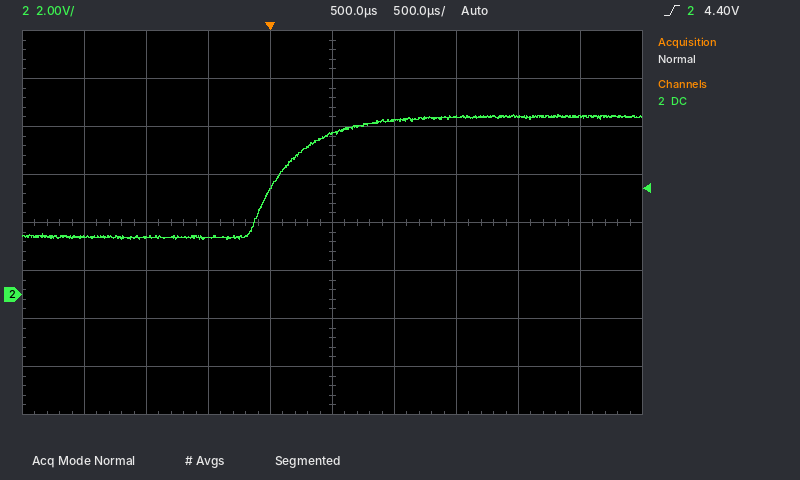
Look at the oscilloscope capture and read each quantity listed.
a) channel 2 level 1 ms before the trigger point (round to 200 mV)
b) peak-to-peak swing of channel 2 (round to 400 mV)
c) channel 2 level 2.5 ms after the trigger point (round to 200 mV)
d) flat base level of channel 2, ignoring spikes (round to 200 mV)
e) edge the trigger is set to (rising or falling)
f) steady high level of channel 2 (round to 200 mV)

2.4 V
5.2 V
7.4 V
2.4 V
rising
7.4 V
